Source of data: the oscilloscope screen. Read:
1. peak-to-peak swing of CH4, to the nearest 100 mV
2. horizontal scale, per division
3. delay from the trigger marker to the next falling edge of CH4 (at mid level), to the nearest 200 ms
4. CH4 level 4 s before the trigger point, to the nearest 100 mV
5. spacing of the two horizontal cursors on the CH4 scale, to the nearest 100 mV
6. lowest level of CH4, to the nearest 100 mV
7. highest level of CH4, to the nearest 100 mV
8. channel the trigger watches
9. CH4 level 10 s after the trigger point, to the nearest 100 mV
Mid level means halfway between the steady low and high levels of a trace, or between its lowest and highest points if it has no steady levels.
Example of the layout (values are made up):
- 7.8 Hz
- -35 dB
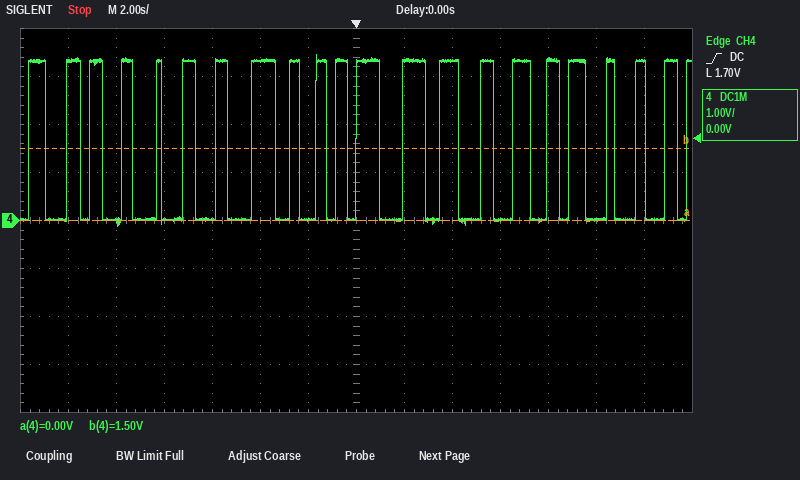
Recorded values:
- 3.6 V
- 2 s
- 1.0 s
- 3.3 V
- 1.5 V
- -100 mV
- 3.5 V
- CH4
- 0.0 V
